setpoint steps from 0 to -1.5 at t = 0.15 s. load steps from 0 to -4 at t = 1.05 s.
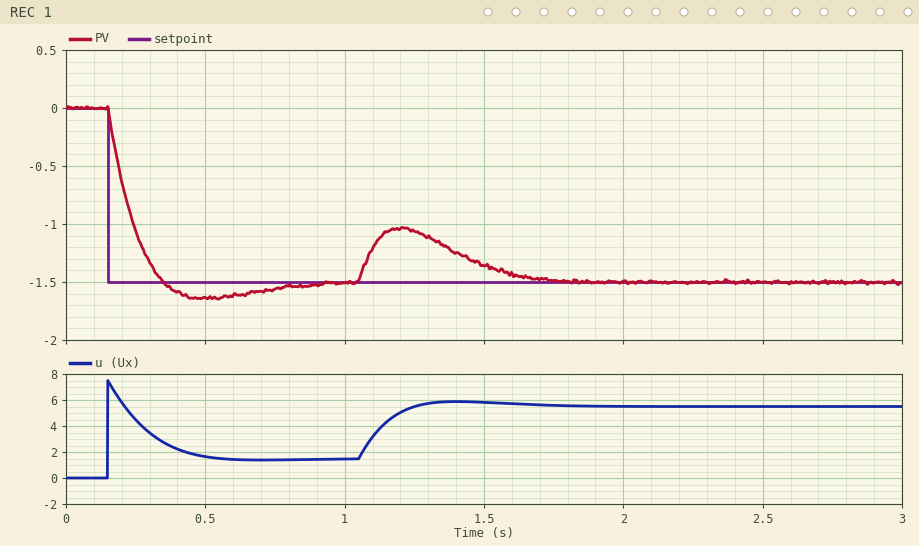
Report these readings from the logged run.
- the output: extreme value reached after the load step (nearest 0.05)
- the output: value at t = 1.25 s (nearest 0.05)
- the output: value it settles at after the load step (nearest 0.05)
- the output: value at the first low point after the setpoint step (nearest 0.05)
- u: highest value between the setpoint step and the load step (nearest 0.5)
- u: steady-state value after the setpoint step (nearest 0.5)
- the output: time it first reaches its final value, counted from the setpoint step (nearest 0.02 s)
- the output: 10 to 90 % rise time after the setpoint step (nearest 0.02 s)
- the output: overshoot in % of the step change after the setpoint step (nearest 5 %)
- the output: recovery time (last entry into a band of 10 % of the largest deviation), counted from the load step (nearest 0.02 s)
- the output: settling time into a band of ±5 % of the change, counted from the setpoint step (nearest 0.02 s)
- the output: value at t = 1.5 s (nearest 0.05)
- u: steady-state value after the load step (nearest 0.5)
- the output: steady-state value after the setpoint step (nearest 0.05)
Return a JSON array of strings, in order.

["-1.05", "-1.05", "-1.50", "-1.65", "7.5", "1.5", "0.20 s", "0.14 s", "10 %", "0.60 s", "0.56 s", "-1.35", "5.5", "-1.50"]
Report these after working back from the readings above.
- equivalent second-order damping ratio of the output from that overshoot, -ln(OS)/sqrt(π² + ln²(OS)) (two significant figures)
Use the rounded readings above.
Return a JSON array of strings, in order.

["0.59"]
